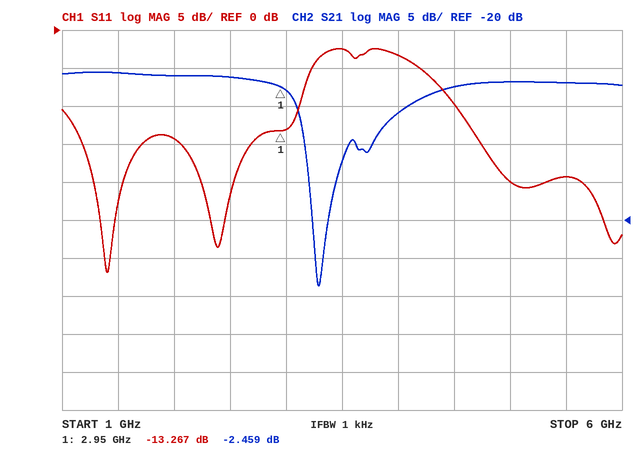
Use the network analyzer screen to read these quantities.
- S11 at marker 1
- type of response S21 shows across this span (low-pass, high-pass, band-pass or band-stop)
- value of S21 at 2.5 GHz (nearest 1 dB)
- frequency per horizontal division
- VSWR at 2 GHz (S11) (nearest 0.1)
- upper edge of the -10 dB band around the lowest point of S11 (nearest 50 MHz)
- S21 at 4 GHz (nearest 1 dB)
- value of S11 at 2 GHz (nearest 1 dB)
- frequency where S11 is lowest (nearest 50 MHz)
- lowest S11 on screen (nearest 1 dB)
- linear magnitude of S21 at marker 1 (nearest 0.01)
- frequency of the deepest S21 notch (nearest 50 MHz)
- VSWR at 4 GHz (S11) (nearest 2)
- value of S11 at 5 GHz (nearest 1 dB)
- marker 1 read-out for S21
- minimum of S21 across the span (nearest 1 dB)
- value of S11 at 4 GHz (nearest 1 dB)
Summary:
-13.267 dB
band-stop
-1 dB
500 MHz
1.5
3.10 GHz
-6 dB
-14 dB
1.40 GHz
-32 dB
0.75
3.30 GHz
6
-20 dB
-2.459 dB
-29 dB
-3 dB
